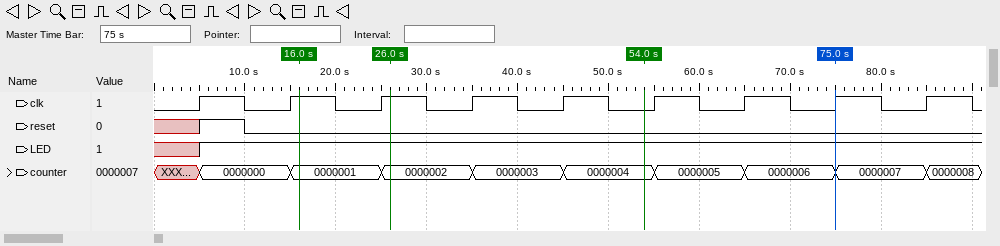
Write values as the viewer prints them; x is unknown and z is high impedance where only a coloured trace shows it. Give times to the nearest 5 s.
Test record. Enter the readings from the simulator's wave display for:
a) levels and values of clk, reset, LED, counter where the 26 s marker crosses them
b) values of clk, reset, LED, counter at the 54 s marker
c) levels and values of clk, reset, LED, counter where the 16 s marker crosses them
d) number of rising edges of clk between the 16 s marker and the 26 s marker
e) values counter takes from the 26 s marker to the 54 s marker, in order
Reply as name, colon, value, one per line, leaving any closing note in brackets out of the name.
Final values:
levels and values of clk, reset, LED, counter where the 26 s marker crosses them: clk=1, reset=0, LED=1, counter=0000002
values of clk, reset, LED, counter at the 54 s marker: clk=0, reset=0, LED=1, counter=0000004
levels and values of clk, reset, LED, counter where the 16 s marker crosses them: clk=1, reset=0, LED=1, counter=0000001
number of rising edges of clk between the 16 s marker and the 26 s marker: 1
values counter takes from the 26 s marker to the 54 s marker, in order: 0000002, 0000003, 0000004
